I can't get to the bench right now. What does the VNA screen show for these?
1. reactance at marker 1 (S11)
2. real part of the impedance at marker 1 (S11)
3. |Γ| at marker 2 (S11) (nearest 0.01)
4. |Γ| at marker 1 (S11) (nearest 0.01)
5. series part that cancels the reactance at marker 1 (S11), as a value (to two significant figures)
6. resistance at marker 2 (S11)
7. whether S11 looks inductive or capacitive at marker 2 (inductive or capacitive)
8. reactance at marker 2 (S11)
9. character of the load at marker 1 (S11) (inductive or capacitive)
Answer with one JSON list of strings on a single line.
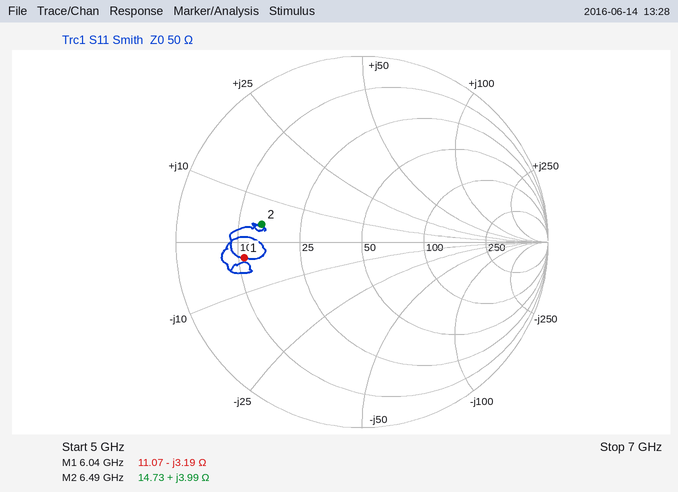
["-3.19 Ω", "11.07 Ω", "0.55", "0.64", "84 pH", "14.73 Ω", "inductive", "+3.99 Ω", "capacitive"]
